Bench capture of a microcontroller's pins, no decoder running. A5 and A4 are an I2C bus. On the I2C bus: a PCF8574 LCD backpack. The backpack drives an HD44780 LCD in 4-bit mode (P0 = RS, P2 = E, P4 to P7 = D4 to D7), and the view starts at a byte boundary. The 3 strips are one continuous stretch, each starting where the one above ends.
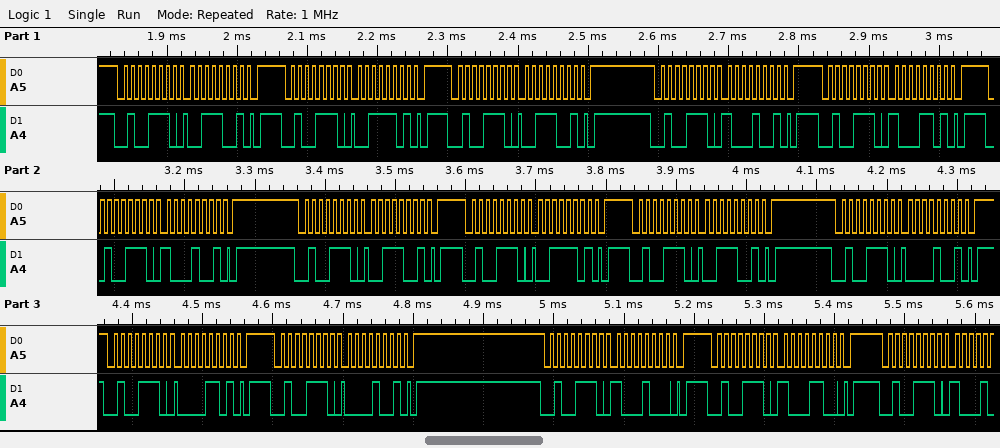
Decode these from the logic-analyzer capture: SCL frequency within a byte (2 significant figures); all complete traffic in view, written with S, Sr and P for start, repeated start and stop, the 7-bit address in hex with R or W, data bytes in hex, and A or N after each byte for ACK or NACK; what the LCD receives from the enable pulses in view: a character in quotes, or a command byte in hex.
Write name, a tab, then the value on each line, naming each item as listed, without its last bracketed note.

SCL frequency within a byte	100 kHz
all complete traffic in view, written with S, Sr and P for start, repeated start and stop, the 7-bit address in hex with R or W, data bytes in hex, and A or N after each byte for ACK or NACK	S 27W A 39 A P S 27W A 3D A P S 27W A 39 A P S 27W A 89 A P S 27W A 8D A P S 27W A 89 A P S 27W A 39 A P S 27W A 3D A P S 27W A 39 A P S 27W A 09 A P S 27W A 0D A P S 27W A 09 A P S 27W A 88 A P S 27W A 8C A P S 27W A
what the LCD receives from the enable pulses in view: a character in quotes, or a command byte in hex	'8' '0'
